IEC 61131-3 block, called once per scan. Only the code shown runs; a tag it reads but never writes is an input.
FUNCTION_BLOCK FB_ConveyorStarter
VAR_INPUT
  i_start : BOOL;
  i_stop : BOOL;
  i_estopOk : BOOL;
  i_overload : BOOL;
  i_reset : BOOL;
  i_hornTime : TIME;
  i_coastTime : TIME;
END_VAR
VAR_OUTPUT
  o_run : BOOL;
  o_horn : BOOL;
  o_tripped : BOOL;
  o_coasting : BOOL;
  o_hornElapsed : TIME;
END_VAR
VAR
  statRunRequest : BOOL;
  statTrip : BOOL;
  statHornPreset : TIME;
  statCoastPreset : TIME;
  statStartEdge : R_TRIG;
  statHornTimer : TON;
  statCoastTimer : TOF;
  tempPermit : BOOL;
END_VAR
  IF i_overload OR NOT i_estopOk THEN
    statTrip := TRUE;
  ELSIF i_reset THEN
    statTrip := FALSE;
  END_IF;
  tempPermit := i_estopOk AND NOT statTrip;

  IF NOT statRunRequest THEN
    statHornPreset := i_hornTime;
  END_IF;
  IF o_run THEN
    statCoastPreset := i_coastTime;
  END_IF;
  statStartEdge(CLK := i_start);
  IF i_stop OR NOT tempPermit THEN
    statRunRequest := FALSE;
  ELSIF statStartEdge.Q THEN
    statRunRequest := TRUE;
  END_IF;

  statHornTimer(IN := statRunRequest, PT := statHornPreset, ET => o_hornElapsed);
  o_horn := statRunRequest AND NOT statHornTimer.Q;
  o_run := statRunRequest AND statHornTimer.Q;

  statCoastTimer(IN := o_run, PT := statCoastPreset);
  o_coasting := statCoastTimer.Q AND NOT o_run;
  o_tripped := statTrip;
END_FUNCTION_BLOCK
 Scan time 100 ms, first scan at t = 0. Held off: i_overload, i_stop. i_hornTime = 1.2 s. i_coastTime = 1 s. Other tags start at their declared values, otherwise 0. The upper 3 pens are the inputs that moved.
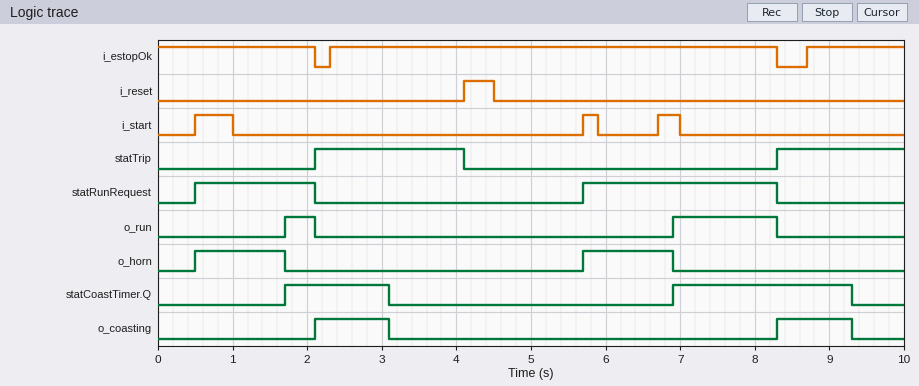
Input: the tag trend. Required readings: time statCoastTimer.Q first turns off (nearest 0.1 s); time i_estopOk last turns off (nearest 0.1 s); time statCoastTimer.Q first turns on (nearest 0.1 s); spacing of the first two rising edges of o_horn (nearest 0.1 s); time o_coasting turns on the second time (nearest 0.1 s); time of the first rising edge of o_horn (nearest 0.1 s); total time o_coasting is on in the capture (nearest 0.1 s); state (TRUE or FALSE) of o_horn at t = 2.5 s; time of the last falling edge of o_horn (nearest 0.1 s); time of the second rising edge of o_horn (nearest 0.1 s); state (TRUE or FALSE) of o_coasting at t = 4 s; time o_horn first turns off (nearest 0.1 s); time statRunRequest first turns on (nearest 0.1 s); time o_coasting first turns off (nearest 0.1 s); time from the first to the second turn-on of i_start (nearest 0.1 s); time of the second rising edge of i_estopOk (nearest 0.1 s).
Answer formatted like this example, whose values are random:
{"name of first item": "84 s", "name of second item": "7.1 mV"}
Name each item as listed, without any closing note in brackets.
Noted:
{"time statCoastTimer.Q first turns off": "3.1 s", "time i_estopOk last turns off": "8.3 s", "time statCoastTimer.Q first turns on": "1.7 s", "spacing of the first two rising edges of o_horn": "5.2 s", "time o_coasting turns on the second time": "8.3 s", "time of the first rising edge of o_horn": "0.5 s", "total time o_coasting is on in the capture": "2.0 s", "state (TRUE or FALSE) of o_horn at t = 2.5 s": "FALSE", "time of the last falling edge of o_horn": "6.9 s", "time of the second rising edge of o_horn": "5.7 s", "state (TRUE or FALSE) of o_coasting at t = 4 s": "FALSE", "time o_horn first turns off": "1.7 s", "time statRunRequest first turns on": "0.5 s", "time o_coasting first turns off": "3.1 s", "time from the first to the second turn-on of i_start": "5.2 s", "time of the second rising edge of i_estopOk": "8.7 s"}
